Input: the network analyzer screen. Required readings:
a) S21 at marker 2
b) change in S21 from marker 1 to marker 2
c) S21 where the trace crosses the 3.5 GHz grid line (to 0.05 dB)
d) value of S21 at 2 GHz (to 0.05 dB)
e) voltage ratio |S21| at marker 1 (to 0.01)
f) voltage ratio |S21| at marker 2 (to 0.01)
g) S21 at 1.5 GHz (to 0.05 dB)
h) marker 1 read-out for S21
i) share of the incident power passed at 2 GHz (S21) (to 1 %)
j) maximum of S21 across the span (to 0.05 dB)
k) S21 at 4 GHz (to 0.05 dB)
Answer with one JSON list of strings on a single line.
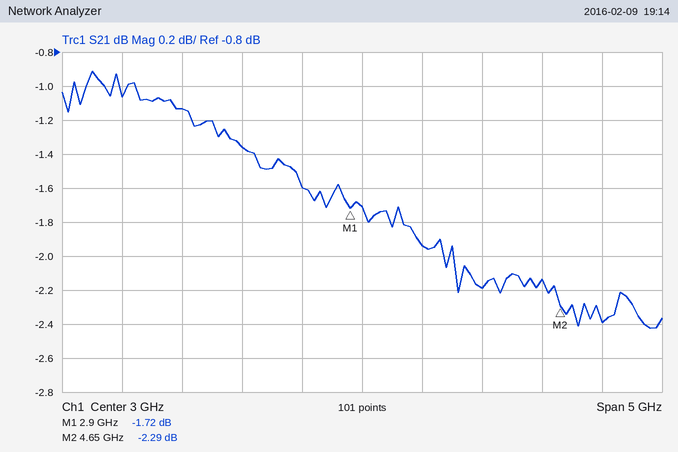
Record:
["-2.29 dB", "-0.57 dB", "-1.95 dB", "-1.35 dB", "0.82", "0.77", "-1.15 dB", "-1.72 dB", "73 %", "-0.90 dB", "-2.20 dB"]
